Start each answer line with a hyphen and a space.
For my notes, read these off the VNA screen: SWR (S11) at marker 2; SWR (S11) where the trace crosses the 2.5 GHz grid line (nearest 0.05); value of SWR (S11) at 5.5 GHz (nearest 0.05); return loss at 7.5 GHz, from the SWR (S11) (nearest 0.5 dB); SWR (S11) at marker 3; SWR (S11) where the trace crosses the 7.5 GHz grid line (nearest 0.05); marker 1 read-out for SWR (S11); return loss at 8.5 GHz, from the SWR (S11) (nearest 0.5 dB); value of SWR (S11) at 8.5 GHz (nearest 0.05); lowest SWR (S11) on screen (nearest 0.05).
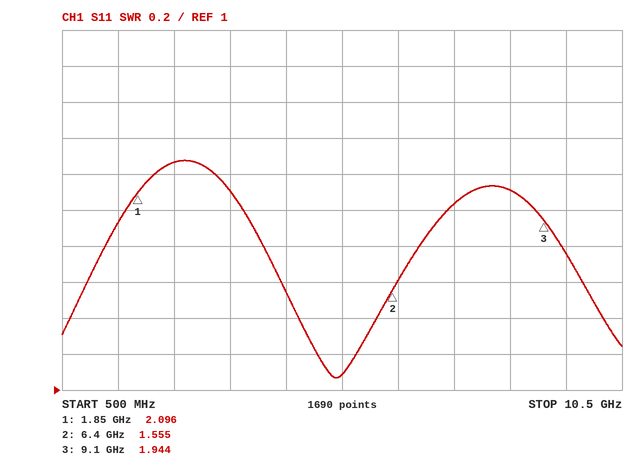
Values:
- 1.555
- 2.25
- 1.10
- 9.5 dB
- 1.944
- 2.05
- 2.096
- 9.0 dB
- 2.10
- 1.05
